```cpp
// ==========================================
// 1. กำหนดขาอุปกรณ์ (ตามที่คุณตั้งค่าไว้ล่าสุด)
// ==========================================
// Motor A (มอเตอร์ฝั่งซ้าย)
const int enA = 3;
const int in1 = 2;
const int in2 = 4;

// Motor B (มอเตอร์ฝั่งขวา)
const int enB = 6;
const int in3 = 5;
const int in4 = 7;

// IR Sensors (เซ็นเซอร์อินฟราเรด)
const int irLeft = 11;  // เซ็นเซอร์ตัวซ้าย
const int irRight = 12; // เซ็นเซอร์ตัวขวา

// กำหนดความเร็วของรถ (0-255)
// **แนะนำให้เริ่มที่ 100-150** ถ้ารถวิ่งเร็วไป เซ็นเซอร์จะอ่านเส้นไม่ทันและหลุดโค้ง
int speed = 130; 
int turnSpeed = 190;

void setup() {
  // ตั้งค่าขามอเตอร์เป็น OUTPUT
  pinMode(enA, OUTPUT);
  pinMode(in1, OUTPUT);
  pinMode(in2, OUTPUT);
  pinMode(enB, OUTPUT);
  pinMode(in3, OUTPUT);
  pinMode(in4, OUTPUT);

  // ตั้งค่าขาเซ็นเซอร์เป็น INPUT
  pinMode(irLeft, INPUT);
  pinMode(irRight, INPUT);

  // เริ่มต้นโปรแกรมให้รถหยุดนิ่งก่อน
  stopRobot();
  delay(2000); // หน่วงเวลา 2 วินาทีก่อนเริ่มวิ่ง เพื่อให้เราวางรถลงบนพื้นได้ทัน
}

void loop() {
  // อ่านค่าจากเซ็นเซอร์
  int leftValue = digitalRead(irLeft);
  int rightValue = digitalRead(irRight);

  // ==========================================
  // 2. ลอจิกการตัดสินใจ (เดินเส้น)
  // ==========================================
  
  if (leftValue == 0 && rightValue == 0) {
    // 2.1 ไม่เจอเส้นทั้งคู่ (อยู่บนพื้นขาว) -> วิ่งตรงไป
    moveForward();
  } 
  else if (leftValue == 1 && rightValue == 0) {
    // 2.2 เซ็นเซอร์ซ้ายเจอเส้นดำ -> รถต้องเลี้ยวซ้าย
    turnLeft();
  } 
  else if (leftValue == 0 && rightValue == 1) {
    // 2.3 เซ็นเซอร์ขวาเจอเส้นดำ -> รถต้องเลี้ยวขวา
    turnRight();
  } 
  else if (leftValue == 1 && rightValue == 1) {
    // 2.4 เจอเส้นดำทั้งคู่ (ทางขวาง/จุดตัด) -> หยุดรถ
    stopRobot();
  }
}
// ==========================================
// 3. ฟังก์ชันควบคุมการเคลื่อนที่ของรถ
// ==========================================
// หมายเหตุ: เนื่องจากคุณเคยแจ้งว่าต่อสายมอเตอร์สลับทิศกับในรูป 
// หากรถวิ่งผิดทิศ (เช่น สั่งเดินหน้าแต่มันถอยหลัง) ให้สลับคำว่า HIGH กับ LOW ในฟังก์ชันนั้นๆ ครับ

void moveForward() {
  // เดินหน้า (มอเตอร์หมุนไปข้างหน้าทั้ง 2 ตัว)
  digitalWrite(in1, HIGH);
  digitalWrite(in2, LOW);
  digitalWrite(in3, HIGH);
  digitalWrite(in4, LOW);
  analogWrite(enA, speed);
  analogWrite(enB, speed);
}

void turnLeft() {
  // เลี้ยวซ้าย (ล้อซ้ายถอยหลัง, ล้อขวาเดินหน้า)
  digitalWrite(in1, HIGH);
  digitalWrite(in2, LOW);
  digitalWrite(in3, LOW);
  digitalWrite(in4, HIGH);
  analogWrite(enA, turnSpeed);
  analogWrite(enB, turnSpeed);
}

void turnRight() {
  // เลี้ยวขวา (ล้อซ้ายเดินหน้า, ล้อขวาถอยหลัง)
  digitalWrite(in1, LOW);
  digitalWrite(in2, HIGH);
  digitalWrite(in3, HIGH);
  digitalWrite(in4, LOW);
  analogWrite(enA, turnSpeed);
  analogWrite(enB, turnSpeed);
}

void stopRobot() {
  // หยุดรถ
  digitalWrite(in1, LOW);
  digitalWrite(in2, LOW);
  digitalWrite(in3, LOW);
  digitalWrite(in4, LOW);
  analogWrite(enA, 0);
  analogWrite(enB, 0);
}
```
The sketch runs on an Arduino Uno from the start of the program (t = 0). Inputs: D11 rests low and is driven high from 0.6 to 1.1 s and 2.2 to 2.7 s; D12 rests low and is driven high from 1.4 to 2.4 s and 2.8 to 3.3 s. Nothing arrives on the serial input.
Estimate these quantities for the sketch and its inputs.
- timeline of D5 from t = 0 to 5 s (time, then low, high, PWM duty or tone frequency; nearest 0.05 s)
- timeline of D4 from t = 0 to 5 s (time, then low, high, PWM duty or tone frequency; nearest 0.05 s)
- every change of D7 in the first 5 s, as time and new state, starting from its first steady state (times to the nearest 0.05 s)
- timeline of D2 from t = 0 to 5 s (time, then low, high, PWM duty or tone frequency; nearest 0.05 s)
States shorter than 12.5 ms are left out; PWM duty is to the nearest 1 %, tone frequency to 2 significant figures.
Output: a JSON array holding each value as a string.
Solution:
["0 s low; 2 s high; 2.2 s low; 2.7 s high", "0 s low; 2 s high; 2.2 s low; 2.8 s high; 3.3 s low", "0 s low; 2.4 s high; 2.7 s low", "0 s low; 2.4 s high; 2.8 s low; 3.3 s high"]
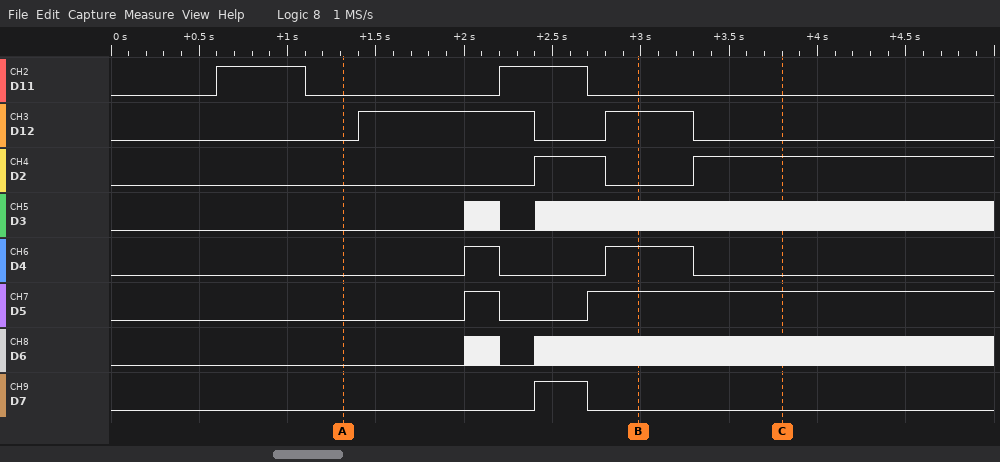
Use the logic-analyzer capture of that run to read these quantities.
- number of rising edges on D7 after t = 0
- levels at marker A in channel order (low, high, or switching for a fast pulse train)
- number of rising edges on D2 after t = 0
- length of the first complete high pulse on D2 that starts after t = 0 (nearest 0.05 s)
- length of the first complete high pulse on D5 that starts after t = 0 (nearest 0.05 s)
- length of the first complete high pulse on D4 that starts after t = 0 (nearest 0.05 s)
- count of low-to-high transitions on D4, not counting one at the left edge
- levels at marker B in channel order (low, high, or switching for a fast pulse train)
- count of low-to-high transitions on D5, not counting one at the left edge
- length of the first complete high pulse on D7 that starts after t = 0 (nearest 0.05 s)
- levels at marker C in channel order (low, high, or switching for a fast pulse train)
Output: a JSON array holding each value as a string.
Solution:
["1", "D11 low, D12 low, D2 low, D3 low, D4 low, D5 low, D6 low, D7 low", "2", "0.40 s", "0.20 s", "0.20 s", "2", "D11 low, D12 high, D2 low, D3 switching, D4 high, D5 high, D6 switching, D7 low", "2", "0.30 s", "D11 low, D12 low, D2 high, D3 switching, D4 low, D5 high, D6 switching, D7 low"]
